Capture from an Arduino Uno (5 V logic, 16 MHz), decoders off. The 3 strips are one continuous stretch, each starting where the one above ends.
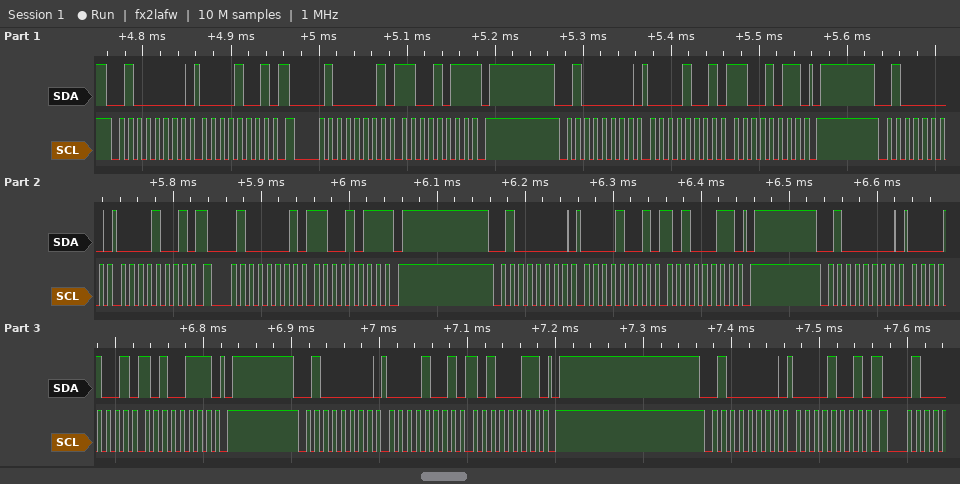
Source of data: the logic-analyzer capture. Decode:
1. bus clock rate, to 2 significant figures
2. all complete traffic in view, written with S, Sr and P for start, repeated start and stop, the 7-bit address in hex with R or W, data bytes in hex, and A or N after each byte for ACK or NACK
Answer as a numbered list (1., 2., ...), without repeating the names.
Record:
1. 100 kHz
2. S 20W A 09 A Sr 20R A CB N P S 20W A 09 A CB A P S 20W A 09 A Sr 20R A CB N P S 20W A 09 A A3 A P S 20W A 09 A A7 A P S 20W A 09 A A3 A P S 20W A 09 A
